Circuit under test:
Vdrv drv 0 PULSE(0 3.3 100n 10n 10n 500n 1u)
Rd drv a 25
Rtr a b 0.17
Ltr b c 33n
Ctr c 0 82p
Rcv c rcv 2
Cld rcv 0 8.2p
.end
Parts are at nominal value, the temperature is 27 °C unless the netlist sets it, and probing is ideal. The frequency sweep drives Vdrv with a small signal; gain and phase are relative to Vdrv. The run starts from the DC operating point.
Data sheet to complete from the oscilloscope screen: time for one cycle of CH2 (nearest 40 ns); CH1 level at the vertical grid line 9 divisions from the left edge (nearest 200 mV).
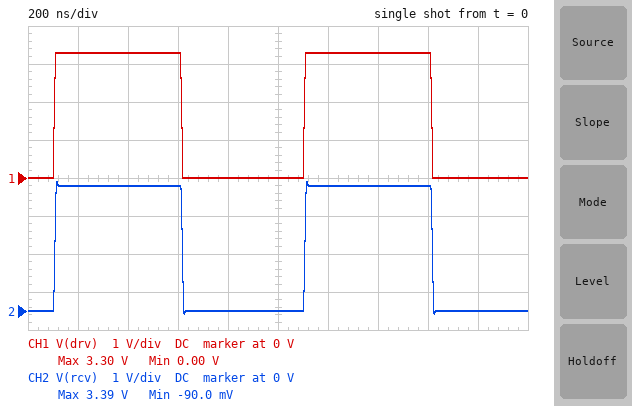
1.00 µs
0 V
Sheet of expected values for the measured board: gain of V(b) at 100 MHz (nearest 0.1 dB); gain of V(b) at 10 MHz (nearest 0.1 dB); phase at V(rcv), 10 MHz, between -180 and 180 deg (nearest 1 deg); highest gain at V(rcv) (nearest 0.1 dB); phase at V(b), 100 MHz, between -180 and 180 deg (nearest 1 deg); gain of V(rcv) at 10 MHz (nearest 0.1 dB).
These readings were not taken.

-18.3 dB
-0.1 dB
-8 deg
0.1 dB
83 deg
0 dB
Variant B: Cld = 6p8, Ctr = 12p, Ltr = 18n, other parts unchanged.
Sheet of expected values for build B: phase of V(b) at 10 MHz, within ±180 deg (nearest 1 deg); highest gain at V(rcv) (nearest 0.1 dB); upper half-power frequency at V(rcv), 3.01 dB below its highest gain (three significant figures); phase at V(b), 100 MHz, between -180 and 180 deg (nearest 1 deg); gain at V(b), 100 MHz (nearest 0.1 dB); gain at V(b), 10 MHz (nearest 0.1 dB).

-2 deg
2.5 dB
325 MHz
-19 deg
-0.5 dB
0 dB
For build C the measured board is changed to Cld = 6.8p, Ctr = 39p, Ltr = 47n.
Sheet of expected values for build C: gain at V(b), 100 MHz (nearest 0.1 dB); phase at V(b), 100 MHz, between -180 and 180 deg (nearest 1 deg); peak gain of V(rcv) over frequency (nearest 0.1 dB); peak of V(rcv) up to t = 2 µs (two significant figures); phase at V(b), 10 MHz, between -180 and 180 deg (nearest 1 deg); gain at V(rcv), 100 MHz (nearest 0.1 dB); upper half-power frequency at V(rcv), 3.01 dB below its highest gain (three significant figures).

-13.9 dB
-78 deg
2.8 dB
3.5 V
-4 deg
2.6 dB
129 MHz
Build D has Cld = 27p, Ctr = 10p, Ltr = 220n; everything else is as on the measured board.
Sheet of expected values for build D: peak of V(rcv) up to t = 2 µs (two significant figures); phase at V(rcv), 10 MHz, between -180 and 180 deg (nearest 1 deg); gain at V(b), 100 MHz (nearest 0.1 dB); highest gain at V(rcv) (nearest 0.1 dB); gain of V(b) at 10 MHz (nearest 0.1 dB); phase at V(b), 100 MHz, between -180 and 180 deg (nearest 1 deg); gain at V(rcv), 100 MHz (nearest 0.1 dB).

4.4 V
-4 deg
-0.3 dB
9.5 dB
0 dB
15 deg
-7.2 dB
